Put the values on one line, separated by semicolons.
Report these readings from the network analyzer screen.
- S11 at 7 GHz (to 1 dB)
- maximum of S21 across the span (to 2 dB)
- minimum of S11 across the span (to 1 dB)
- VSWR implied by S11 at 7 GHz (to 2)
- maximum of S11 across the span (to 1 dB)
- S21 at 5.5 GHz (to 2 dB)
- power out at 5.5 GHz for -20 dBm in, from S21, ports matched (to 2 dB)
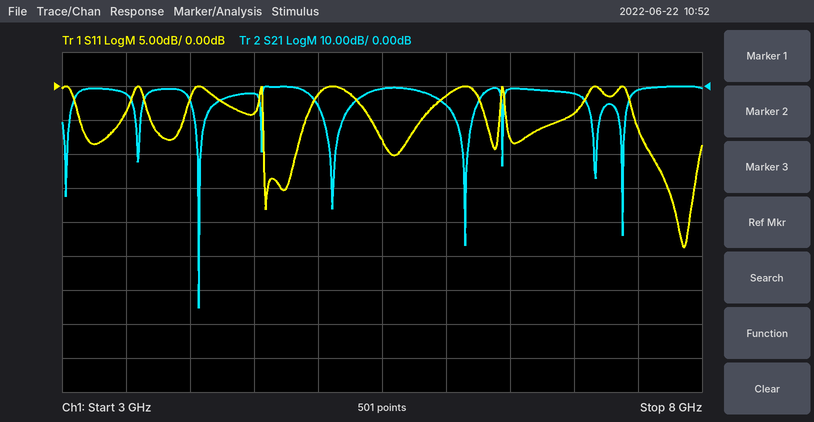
-4 dB; 0 dB; -24 dB; 4; 0 dB; 0 dB; -20 dBm
